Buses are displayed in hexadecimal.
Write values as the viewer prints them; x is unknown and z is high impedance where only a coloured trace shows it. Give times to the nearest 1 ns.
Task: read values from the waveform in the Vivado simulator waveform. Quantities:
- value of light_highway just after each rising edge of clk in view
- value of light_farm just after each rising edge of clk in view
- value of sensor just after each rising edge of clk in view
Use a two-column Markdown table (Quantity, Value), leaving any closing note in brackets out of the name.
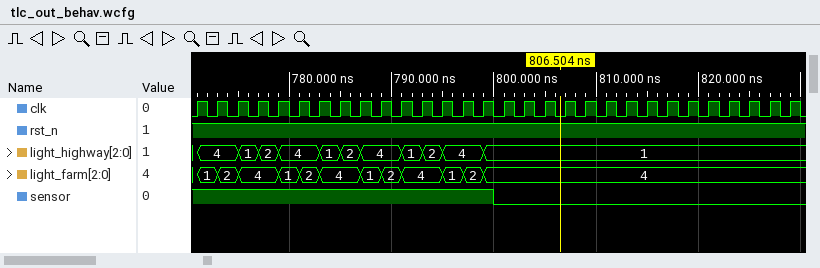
| Quantity | Value |
|---|---|
| value of light_highway just after each rising edge of clk in view | 4, 4, 1, 2, 4, 4, 1, 2, 4, 4, 1, 2, 4, 4, 1, 1, 1, 1, 1, 1, 1, 1, 1, 1, 1, 1, 1, 1, 1, 1 |
| value of light_farm just after each rising edge of clk in view | 1, 2, 4, 4, 1, 2, 4, 4, 1, 2, 4, 4, 1, 2, 4, 4, 4, 4, 4, 4, 4, 4, 4, 4, 4, 4, 4, 4, 4, 4 |
| value of sensor just after each rising edge of clk in view | 1 1 1 1 1 1 1 1 1 1 1 1 1 1 1 0 0 0 0 0 0 0 0 0 0 0 0 0 0 0 |
